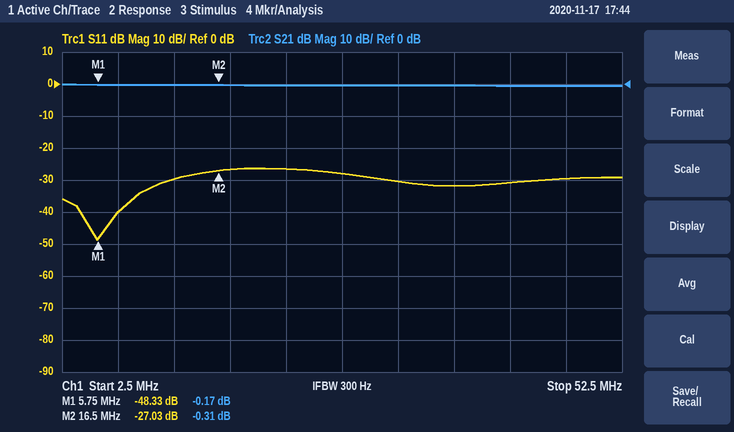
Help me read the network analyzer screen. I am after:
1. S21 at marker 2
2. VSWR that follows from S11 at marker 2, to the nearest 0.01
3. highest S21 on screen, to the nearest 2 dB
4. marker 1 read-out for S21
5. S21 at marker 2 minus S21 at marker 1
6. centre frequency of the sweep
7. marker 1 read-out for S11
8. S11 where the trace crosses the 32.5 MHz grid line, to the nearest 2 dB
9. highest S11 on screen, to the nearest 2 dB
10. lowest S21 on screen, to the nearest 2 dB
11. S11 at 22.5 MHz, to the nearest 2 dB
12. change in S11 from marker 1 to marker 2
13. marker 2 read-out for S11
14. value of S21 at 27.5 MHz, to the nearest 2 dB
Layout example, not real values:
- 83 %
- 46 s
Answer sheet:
- -0.31 dB
- 1.09
- 0 dB
- -0.17 dB
- -0.14 dB
- 27.5 MHz
- -48.33 dB
- -30 dB
- -26 dB
- 0 dB
- -26 dB
- 21.30 dB
- -27.03 dB
- 0 dB
